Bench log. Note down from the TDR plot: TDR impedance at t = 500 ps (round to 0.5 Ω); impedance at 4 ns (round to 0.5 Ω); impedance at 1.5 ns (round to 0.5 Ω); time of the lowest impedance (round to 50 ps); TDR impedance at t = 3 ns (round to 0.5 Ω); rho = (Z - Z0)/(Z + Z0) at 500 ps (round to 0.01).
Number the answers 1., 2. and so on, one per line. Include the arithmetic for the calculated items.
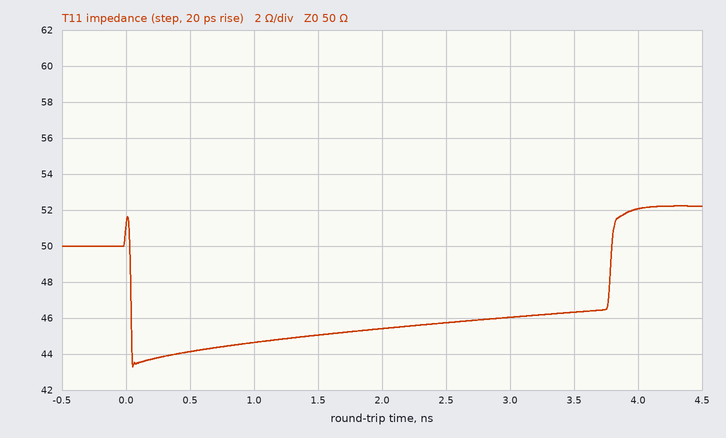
1. 44.0 Ω
2. 52.0 Ω
3. 45.0 Ω
4. 50 ps
5. 46.0 Ω
6. (44 − 50)/(44 + 50) ≈ -0.06
